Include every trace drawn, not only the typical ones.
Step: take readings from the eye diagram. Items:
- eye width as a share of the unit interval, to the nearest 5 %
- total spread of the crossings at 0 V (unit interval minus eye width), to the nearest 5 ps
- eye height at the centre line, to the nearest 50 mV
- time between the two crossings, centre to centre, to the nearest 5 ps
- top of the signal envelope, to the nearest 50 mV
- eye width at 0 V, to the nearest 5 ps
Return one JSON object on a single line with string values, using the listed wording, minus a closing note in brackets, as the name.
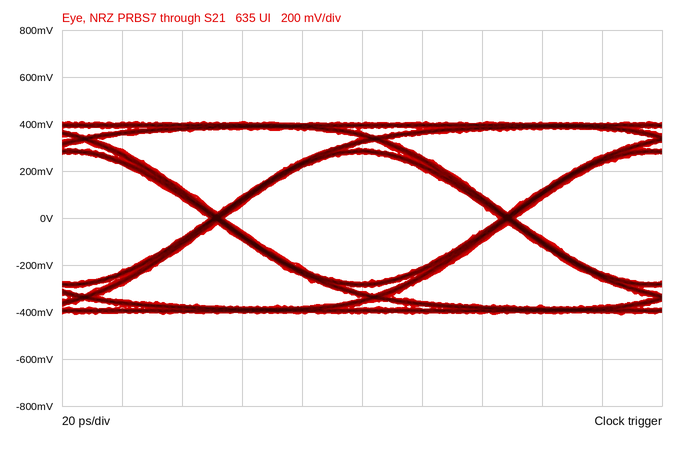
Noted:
{"eye width as a share of the unit interval, to the nearest 5 %": "95 %", "total spread of the crossings at 0 V (unit interval minus eye width), to the nearest 5 ps": "5 ps", "eye height at the centre line, to the nearest 50 mV": "550 mV", "time between the two crossings, centre to centre, to the nearest 5 ps": "95 ps", "top of the signal envelope, to the nearest 50 mV": "400 mV", "eye width at 0 V, to the nearest 5 ps": "90 ps"}
